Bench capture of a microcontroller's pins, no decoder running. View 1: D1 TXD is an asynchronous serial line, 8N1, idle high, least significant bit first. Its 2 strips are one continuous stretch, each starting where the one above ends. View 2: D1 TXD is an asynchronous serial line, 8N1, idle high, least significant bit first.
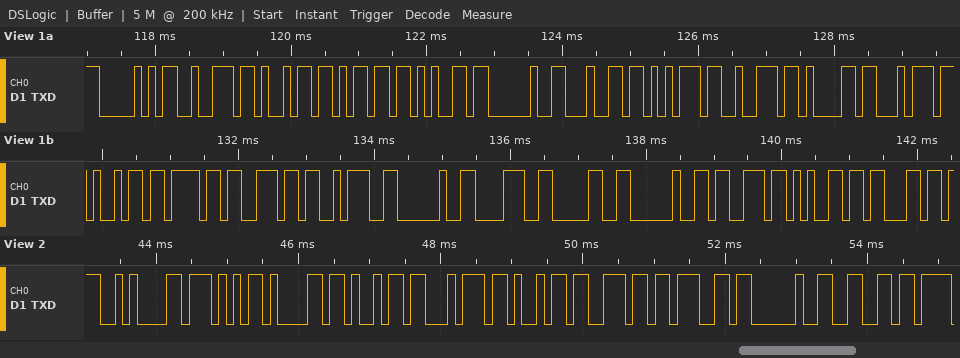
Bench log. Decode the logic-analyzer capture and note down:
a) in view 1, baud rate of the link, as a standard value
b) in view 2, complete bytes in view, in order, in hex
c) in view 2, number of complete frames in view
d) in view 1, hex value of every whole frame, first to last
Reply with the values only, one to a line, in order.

9600 baud
0A 57 61 69 74 69 6E 67 20 66
10
50 72 69 6D 65 20 64 75 72 61 74 69 6F 6E 3A 20 38 30 20 73 65 63
